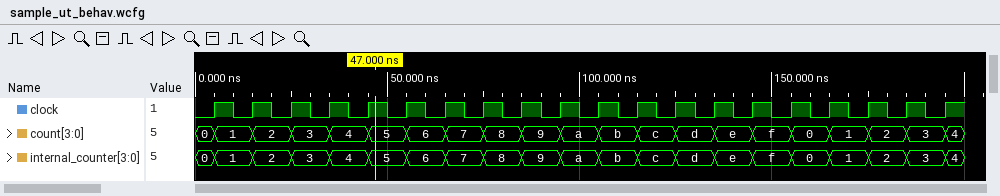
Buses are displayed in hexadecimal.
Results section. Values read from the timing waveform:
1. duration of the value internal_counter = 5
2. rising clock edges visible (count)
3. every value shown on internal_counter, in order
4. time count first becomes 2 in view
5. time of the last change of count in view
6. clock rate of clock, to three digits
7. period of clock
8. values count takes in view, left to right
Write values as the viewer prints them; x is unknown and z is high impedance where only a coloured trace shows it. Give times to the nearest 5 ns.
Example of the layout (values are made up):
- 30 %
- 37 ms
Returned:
- 10 ns
- 20
- 0, 1, 2, 3, 4, 5, 6, 7, 8, 9, a, b, c, d, e, f, 0, 1, 2, 3, 4
- 15 ns
- 195 ns
- 100 MHz
- 10 ns
- 0, 1, 2, 3, 4, 5, 6, 7, 8, 9, a, b, c, d, e, f, 0, 1, 2, 3, 4
